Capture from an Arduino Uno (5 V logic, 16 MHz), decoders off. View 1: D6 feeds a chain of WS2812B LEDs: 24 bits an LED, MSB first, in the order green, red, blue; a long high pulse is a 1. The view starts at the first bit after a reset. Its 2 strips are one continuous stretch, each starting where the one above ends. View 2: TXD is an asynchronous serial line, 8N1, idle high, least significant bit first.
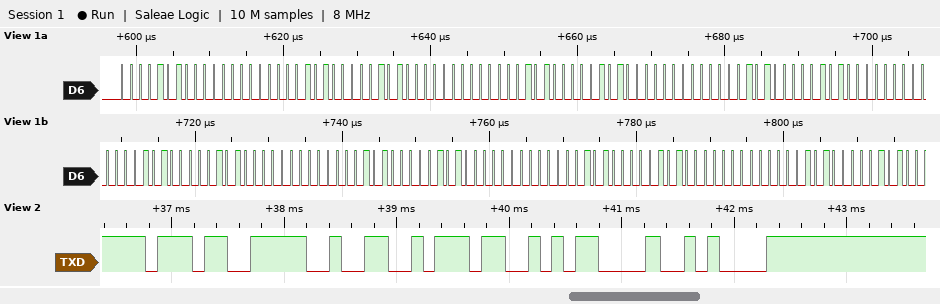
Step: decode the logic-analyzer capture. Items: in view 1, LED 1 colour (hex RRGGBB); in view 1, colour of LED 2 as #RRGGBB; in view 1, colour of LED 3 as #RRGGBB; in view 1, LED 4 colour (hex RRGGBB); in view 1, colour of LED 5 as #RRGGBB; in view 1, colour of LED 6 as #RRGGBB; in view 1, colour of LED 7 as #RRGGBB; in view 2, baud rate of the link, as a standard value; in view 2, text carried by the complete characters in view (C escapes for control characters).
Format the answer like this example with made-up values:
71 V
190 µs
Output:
#000A0A
#000A0A
#000A0A
#000A0A
#000A0A
#000A0A
#000A0A
9600 baud
"727\r\n"
